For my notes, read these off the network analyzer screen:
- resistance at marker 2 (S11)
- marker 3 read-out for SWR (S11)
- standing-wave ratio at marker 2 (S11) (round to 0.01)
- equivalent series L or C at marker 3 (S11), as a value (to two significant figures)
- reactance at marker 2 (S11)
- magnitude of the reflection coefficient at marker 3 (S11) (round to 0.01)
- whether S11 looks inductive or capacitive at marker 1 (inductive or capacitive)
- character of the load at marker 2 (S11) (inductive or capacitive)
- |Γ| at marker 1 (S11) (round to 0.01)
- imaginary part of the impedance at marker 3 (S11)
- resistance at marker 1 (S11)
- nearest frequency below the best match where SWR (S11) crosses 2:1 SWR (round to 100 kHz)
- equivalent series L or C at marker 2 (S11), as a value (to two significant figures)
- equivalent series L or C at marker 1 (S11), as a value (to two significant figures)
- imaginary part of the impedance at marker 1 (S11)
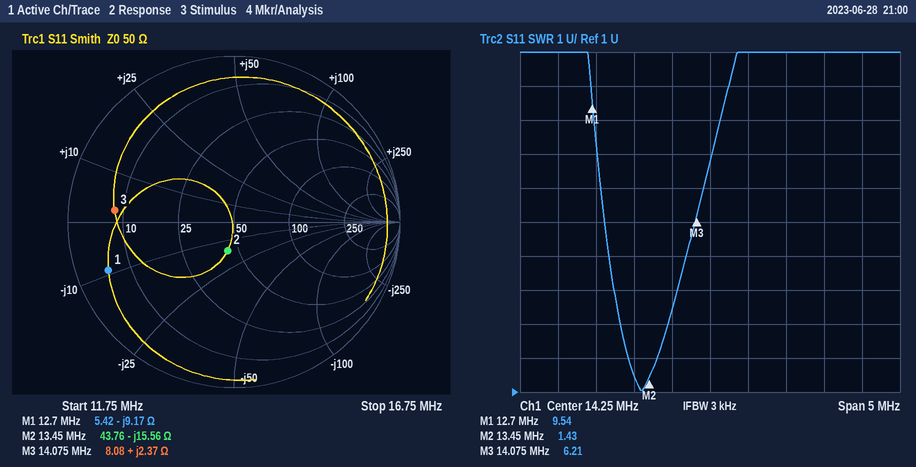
43.76 Ω
6.21
1.43
27 nH
-15.56 Ω
0.72
capacitive
capacitive
0.81
+2.37 Ω
5.42 Ω
13.2 MHz
760 pF
1.4 nF
-9.17 Ω
